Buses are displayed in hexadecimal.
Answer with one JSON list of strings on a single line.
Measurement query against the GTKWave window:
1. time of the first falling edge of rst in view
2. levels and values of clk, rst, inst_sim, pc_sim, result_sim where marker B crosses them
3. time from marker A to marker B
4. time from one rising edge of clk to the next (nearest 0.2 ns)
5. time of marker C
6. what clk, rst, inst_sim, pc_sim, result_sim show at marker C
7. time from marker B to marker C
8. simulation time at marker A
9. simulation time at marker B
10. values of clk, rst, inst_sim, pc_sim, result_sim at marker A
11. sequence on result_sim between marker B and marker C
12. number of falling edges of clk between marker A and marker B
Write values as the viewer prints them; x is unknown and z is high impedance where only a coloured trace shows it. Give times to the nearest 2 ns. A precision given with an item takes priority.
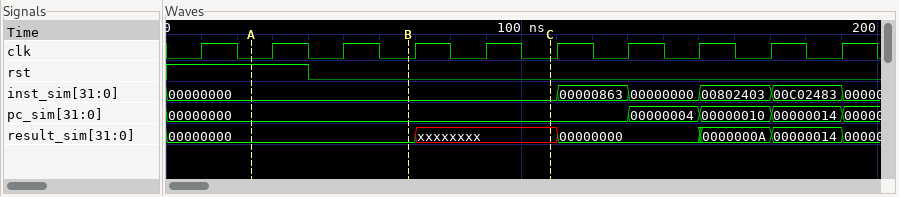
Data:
["40 ns", "clk=0, rst=0, inst_sim=00000000, pc_sim=00000000, result_sim=00000000", "44 ns", "20 ns", "108 ns", "clk=0, rst=0, inst_sim=00000000, pc_sim=00000000, result_sim=xxxxxxxx", "40 ns", "24 ns", "68 ns", "clk=0, rst=1, inst_sim=00000000, pc_sim=00000000, result_sim=00000000", "00000000, xxxxxxxx", "2"]
